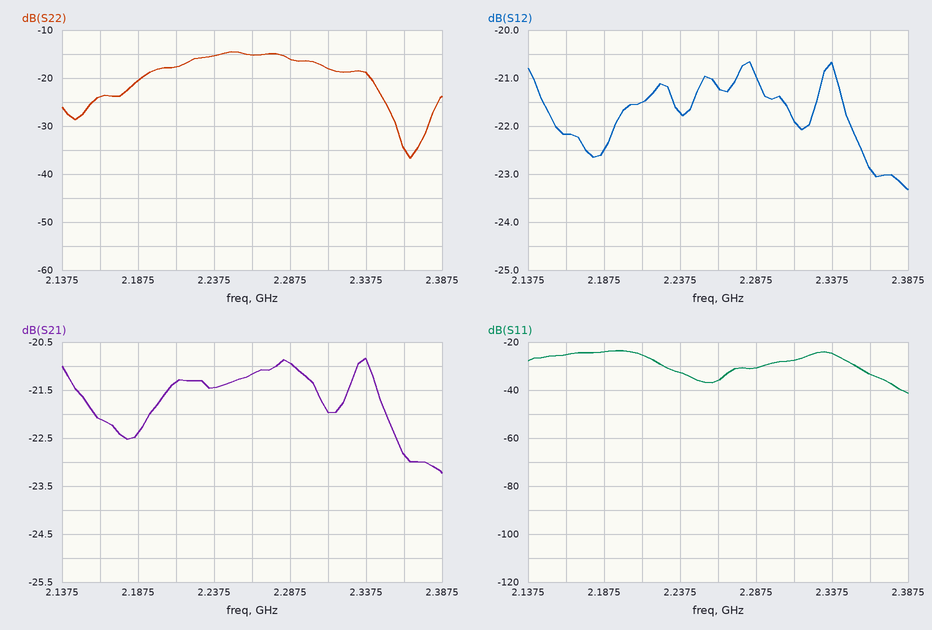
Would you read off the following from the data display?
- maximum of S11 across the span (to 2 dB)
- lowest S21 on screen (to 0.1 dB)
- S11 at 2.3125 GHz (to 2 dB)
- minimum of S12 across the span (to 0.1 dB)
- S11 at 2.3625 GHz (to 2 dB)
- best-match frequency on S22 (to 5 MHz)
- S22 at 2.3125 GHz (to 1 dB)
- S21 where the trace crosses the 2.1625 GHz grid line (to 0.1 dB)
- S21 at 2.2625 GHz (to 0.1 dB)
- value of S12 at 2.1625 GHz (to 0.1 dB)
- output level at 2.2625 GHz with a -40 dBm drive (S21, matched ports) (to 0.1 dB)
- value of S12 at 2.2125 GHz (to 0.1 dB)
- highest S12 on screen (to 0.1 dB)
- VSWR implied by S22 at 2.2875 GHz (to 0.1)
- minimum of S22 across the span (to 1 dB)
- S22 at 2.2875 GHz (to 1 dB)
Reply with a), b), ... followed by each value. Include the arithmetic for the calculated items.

a) -24 dB
b) -23.2 dB
c) -28 dB
d) -23.3 dB
e) -34 dB
f) 2.365 GHz
g) -18 dB
h) -22.1 dB
i) -21.2 dB
j) -22.2 dB
k) -40 dBm + (-21.2 dB) = -61.2 dBm
l) -21.5 dB
m) -20.7 dB
n) |Γ| = 10^(-16/20) = 0.1585; VSWR = (1 + 0.1585)/(1 − 0.1585) ≈ 1.4
o) -37 dB
p) -16 dB
